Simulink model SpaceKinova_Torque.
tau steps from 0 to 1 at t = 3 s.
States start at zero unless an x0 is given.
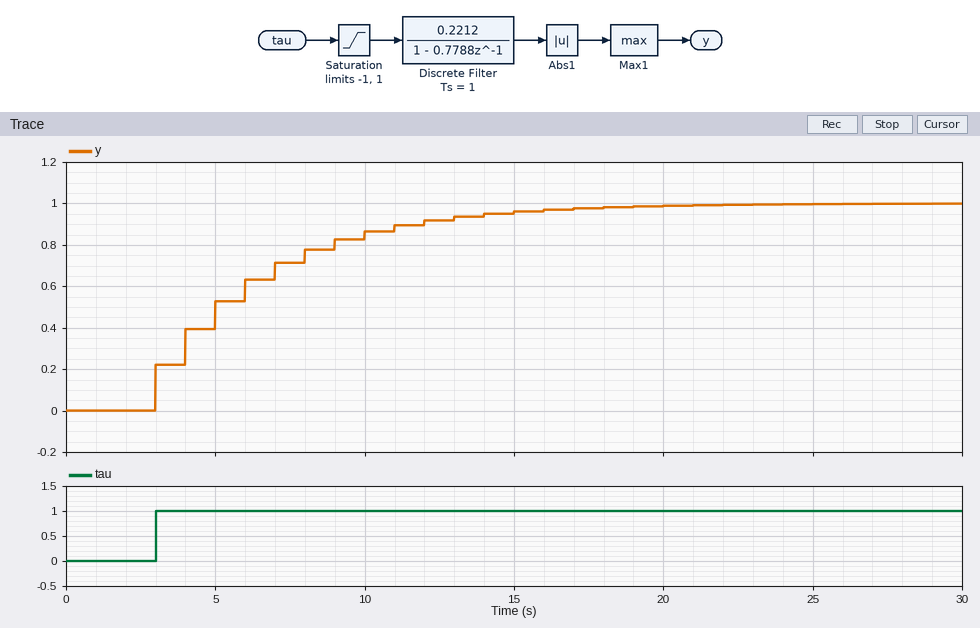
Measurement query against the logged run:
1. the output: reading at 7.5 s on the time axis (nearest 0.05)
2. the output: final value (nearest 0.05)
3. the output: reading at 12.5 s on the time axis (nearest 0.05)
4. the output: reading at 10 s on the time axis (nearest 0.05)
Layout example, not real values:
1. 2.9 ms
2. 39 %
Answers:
1. 0.70
2. 1.00
3. 0.90
4. 0.85
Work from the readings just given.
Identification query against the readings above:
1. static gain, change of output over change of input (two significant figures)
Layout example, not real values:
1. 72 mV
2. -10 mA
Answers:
1. 1.0
